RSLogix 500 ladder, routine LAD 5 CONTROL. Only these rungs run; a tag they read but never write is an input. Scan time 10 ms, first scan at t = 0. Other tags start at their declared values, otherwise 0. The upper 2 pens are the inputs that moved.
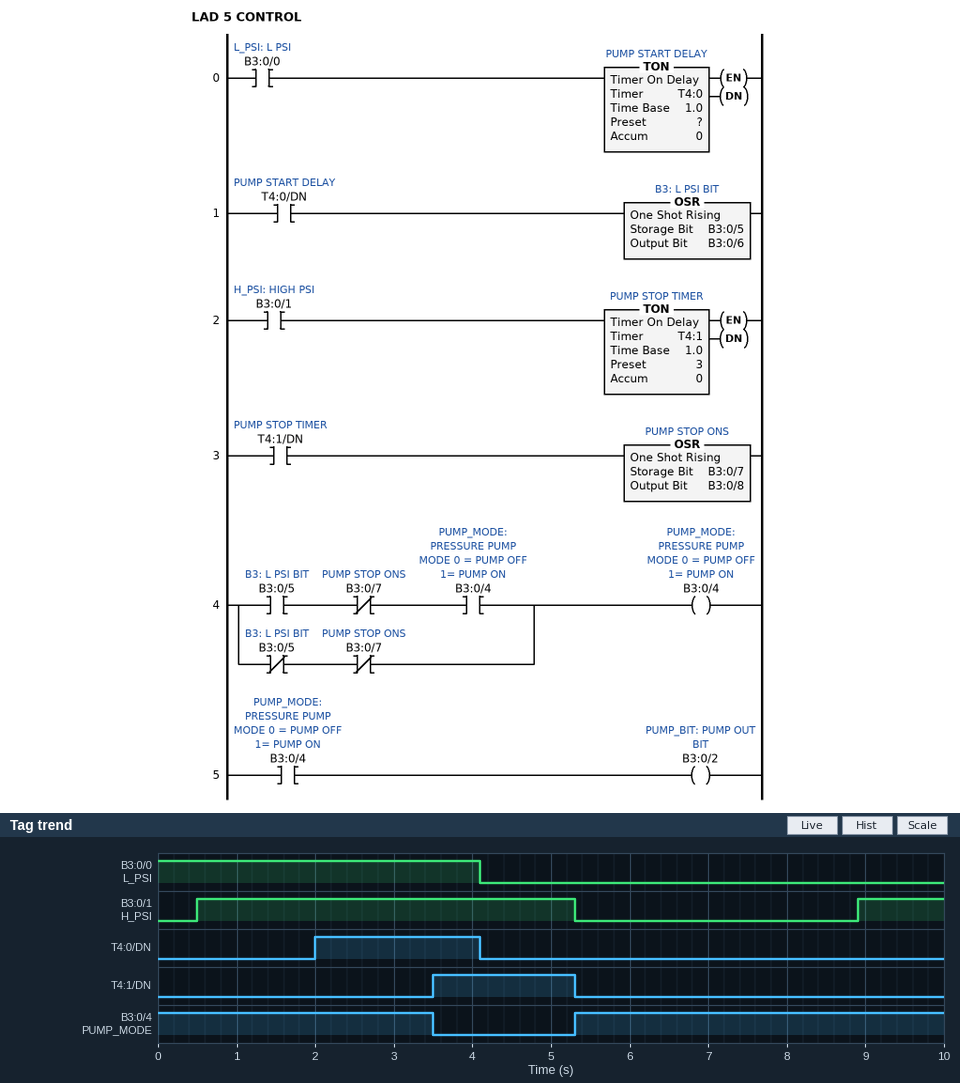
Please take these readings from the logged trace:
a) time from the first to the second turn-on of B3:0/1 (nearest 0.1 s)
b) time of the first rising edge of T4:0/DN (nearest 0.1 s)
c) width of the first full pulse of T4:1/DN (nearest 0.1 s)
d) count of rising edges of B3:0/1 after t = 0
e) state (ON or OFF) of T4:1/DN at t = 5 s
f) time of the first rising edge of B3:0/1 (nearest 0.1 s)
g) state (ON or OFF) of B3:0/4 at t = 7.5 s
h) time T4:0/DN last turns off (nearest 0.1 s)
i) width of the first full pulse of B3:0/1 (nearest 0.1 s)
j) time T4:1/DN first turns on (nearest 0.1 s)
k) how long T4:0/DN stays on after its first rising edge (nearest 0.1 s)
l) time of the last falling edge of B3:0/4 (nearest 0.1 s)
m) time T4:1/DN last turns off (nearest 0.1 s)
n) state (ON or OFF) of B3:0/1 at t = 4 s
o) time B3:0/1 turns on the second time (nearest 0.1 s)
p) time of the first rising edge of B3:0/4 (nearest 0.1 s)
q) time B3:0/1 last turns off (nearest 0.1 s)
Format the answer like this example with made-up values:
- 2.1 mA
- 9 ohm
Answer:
- 8.4 s
- 2.0 s
- 1.8 s
- 2
- ON
- 0.5 s
- ON
- 4.1 s
- 4.8 s
- 3.5 s
- 2.1 s
- 3.5 s
- 5.3 s
- ON
- 8.9 s
- 5.3 s
- 5.3 s
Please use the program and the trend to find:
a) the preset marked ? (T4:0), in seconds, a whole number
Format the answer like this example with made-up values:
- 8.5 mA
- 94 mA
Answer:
- 2 s
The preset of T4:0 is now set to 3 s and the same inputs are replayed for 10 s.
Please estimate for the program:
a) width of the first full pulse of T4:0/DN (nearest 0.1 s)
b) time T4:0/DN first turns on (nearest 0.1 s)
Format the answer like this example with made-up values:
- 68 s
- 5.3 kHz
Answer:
- 1.1 s
- 3.0 s
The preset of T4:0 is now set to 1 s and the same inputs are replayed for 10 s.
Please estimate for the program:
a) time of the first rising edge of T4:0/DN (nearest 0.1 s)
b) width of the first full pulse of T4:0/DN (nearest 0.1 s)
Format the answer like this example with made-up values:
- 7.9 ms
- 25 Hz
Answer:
- 1.0 s
- 3.1 s
